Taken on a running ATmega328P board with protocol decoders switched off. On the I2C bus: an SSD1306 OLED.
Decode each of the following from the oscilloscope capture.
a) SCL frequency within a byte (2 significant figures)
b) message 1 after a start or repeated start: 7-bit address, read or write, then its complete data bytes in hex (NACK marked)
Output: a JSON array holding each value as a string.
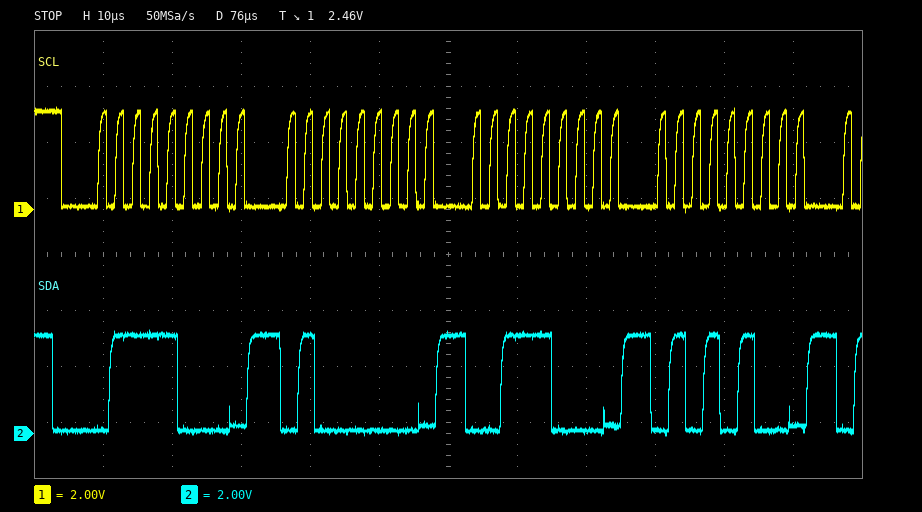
["400 kHz", "0x3C write: 40 38 54"]
